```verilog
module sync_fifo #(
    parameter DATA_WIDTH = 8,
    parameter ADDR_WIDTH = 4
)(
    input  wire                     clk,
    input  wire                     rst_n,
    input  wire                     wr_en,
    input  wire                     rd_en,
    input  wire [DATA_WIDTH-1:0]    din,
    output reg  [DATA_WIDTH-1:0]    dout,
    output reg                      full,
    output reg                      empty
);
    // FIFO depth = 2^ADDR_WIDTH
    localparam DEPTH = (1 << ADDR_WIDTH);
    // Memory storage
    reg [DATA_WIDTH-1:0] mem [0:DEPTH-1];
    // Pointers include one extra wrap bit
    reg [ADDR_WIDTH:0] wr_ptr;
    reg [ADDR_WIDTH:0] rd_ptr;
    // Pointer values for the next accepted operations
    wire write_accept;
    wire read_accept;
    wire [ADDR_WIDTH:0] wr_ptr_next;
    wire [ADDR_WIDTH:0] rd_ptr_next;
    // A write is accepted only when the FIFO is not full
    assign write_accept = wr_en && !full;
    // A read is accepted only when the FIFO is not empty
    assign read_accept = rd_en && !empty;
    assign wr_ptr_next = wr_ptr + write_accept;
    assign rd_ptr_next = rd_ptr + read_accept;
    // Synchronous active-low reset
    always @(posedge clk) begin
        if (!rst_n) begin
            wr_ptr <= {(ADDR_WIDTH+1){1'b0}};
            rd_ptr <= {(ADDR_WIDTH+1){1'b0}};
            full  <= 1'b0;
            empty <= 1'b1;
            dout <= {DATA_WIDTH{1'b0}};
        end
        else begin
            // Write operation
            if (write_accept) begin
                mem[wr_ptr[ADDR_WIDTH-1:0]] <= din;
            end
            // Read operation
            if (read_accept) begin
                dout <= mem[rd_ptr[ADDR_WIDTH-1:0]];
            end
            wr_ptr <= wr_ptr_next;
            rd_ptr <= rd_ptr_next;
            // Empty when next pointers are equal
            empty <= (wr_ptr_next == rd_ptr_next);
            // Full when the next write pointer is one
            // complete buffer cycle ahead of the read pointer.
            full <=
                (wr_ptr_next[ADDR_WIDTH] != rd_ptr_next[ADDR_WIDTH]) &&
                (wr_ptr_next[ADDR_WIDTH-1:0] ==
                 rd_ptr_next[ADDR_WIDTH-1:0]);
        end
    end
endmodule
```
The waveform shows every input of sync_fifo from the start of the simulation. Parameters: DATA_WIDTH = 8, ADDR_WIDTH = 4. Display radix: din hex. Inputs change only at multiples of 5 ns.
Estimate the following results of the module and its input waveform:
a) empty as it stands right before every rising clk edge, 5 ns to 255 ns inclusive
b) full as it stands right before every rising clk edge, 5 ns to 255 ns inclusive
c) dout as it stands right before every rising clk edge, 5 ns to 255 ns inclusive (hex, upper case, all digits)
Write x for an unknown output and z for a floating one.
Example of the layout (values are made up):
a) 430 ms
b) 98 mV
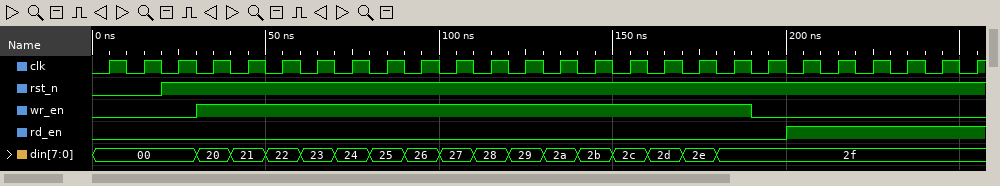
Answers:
a) x 1 1 1 0 0 0 0 0 0 0 0 0 0 0 0 0 0 0 0 0 0 0 0 0 0
b) x 0 0 0 0 0 0 0 0 0 0 0 0 0 0 0 0 0 0 1 1 0 0 0 0 0
c) x, 00, 00, 00, 00, 00, 00, 00, 00, 00, 00, 00, 00, 00, 00, 00, 00, 00, 00, 00, 00, 20, 21, 22, 23, 24
